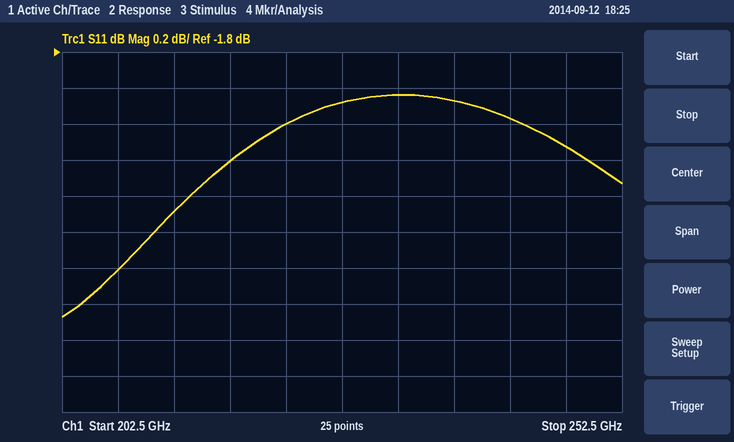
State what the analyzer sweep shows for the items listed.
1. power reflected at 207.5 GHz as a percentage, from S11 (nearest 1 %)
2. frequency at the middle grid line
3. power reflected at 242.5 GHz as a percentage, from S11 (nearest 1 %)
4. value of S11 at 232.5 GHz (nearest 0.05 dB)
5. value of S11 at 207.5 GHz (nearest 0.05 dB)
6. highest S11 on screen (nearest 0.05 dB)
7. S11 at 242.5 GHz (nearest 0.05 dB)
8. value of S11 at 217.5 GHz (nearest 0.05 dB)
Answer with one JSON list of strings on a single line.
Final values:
["50 %", "227.5 GHz", "61 %", "-2.05 dB", "-3.00 dB", "-2.05 dB", "-2.15 dB", "-2.40 dB"]
